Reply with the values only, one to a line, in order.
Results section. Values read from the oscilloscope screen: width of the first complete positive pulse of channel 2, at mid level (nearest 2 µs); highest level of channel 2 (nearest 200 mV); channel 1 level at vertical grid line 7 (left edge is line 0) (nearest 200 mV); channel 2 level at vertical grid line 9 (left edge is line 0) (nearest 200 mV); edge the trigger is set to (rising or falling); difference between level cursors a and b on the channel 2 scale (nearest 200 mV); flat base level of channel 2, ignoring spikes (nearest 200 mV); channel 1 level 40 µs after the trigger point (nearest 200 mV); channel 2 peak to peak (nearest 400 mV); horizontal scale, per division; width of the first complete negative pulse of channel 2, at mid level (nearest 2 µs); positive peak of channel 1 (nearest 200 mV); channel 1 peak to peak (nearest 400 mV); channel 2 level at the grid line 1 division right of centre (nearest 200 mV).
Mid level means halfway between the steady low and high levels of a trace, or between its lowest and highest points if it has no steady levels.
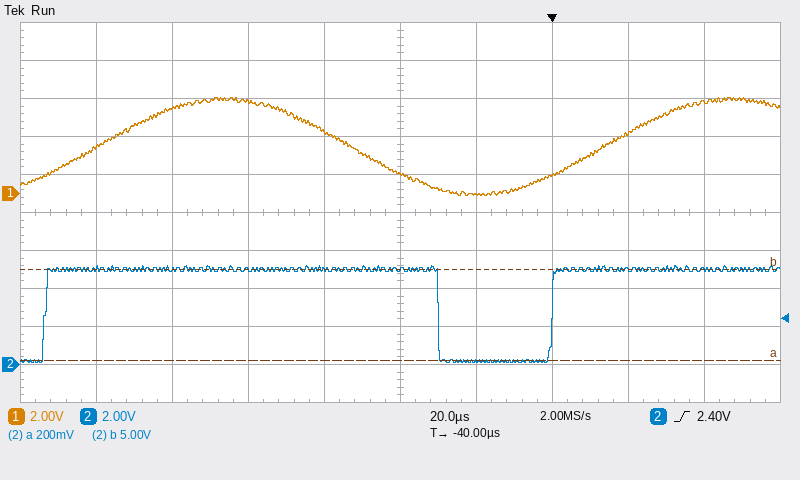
104 µs
5.2 V
1.0 V
5.0 V
rising
4.8 V
200 mV
4.8 V
5.2 V
20 µs
30 µs
5.0 V
5.2 V
200 mV
